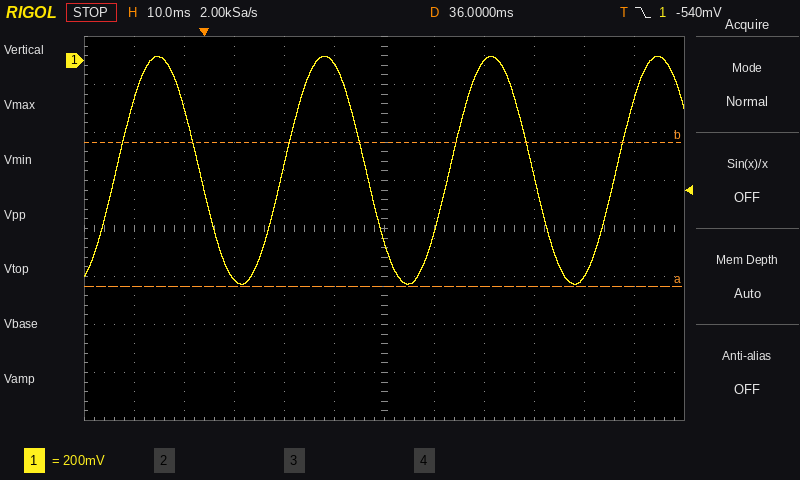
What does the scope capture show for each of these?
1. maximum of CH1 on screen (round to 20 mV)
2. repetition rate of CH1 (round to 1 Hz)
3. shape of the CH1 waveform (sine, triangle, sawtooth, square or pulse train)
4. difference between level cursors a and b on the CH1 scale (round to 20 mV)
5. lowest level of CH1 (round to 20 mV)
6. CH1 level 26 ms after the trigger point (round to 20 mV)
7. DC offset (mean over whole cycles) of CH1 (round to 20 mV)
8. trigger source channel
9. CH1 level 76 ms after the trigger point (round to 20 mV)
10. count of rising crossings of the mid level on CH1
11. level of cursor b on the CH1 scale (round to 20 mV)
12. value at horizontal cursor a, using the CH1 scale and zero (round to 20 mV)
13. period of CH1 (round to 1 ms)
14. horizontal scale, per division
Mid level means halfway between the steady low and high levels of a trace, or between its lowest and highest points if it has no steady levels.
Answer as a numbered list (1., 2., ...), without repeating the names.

1. 20 mV
2. 30 Hz
3. sine
4. 600 mV
5. -940 mV
6. -20 mV
7. -460 mV
8. CH1
9. -900 mV
10. 4
11. -340 mV
12. -940 mV
13. 33 ms
14. 10 ms
